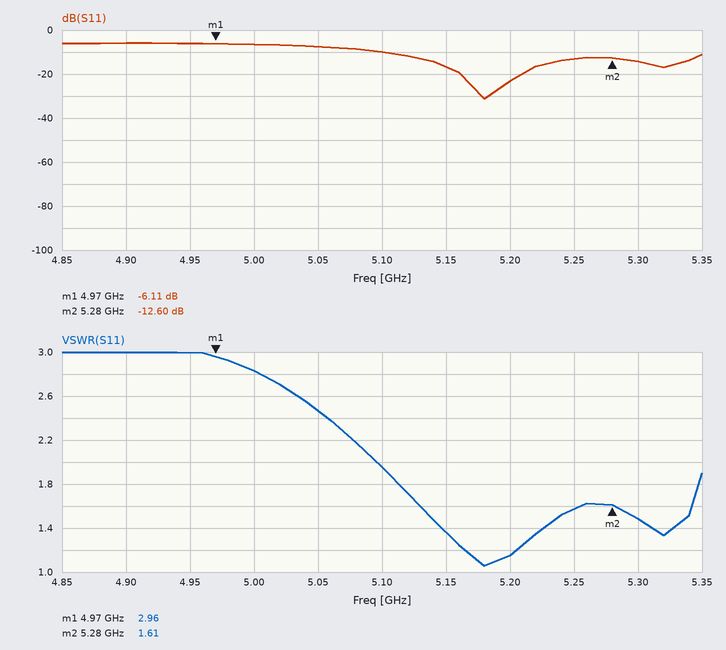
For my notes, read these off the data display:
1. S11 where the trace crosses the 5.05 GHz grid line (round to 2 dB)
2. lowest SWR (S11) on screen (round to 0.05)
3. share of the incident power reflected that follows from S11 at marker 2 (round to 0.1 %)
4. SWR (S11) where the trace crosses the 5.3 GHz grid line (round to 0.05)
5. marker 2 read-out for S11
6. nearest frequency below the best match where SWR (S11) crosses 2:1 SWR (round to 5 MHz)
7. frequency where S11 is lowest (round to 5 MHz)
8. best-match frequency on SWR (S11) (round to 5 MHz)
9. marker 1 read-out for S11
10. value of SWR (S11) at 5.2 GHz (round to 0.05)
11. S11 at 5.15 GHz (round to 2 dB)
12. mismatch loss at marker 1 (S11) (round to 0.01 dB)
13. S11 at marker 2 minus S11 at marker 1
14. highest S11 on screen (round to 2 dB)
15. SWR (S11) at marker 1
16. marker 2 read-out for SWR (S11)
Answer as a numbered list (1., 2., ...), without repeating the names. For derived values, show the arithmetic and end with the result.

1. -8 dB
2. 1.05
3. 10^(-12.6/10) ≈ 5.5 %
4. 1.50
5. -12.60 dB
6. 5.095 GHz
7. 5.180 GHz
8. 5.180 GHz
9. -6.11 dB
10. 1.15
11. -16 dB
12. −10 log10(1 − 10^(-6.11/10)) ≈ 1.22 dB
13. -12.6 − (-6.11) = -6.49 dB
14. -6 dB
15. 2.96
16. 1.61
